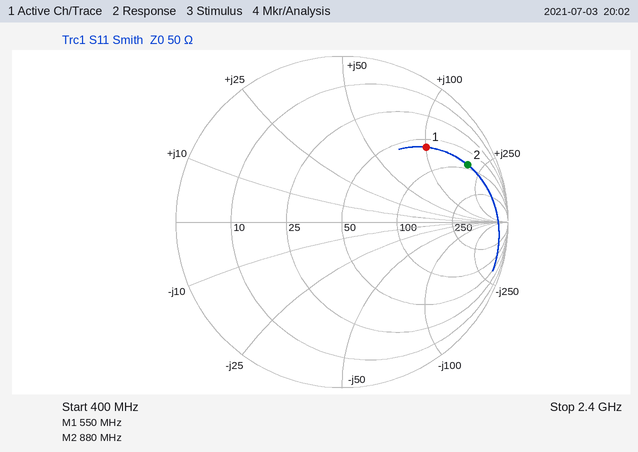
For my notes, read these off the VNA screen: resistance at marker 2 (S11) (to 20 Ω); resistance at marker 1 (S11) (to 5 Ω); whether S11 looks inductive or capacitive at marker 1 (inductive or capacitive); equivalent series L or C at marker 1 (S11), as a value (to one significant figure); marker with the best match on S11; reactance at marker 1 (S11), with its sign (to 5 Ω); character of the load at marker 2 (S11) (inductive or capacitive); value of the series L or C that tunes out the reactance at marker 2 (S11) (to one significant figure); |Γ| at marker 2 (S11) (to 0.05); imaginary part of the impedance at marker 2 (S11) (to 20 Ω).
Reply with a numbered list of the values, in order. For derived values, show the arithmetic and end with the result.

1. 80 Ω
2. 60 Ω
3. inductive
4. L = 100 Ω/(2π × 550 MHz) ≈ 28.9 nH, so 30 nH to one significant figure
5. marker 1
6. +100 Ω
7. inductive
8. C = 1/(2π × 880 MHz × 200 Ω) ≈ 904 fF, so 900 fF to one significant figure
9. 0.85
10. +200 Ω
